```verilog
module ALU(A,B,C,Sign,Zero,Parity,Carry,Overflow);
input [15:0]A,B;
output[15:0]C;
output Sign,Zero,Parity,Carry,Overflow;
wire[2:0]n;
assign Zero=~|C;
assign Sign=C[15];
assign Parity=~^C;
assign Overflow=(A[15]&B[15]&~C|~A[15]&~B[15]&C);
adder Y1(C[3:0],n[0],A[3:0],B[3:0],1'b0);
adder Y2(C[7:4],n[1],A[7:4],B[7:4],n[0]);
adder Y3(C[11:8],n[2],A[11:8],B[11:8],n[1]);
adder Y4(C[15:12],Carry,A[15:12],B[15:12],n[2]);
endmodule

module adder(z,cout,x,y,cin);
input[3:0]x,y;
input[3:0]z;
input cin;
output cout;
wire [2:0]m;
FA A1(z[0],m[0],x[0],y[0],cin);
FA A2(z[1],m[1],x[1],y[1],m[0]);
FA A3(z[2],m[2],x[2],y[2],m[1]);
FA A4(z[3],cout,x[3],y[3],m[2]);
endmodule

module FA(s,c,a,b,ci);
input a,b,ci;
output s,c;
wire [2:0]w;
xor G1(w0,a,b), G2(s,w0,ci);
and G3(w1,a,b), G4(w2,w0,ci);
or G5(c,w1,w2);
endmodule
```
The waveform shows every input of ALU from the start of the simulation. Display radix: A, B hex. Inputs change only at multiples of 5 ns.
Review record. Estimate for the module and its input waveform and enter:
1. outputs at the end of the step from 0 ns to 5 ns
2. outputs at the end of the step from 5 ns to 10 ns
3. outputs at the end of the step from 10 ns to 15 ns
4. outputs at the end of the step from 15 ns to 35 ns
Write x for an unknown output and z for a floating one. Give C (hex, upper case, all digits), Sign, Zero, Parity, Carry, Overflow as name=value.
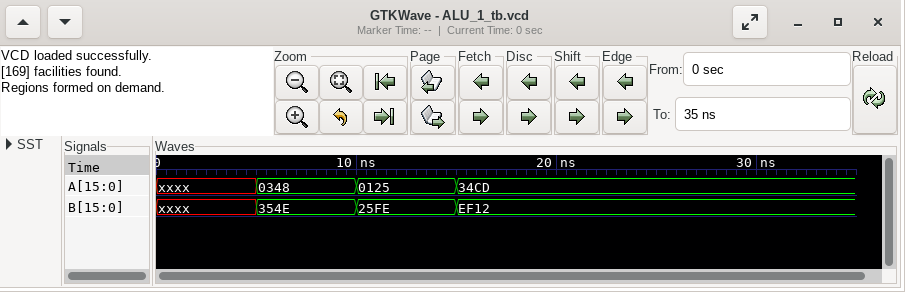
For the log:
C=x, Sign=x, Zero=x, Parity=x, Carry=x, Overflow=x
C=3896, Sign=0, Zero=0, Parity=0, Carry=0, Overflow=0
C=2723, Sign=0, Zero=0, Parity=0, Carry=0, Overflow=1
C=23DF, Sign=0, Zero=0, Parity=1, Carry=1, Overflow=0
